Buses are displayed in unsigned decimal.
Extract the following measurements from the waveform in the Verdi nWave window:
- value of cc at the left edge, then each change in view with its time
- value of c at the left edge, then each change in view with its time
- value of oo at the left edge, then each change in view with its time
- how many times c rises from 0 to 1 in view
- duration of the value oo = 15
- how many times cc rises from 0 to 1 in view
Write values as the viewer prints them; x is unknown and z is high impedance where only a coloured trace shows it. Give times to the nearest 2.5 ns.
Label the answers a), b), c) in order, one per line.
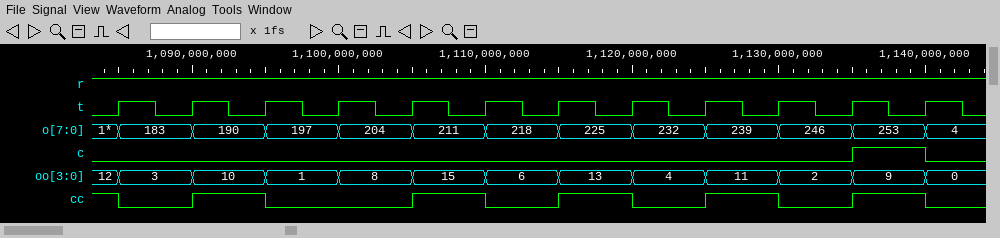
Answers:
a) 1, 0 at 1085 ns, 1 at 1090 ns, 0 at 1095 ns, 1 at 1105 ns, 0 at 1110 ns, 1 at 1115 ns, 0 at 1120 ns, 1 at 1125 ns, 0 at 1130 ns, 1 at 1135 ns, 0 at 1140 ns
b) 0, 1 at 1135 ns, 0 at 1140 ns
c) 12, 3 at 1085 ns, 10 at 1090 ns, 1 at 1095 ns, 8 at 1100 ns, 15 at 1105 ns, 6 at 1110 ns, 13 at 1115 ns, 4 at 1120 ns, 11 at 1125 ns, 2 at 1130 ns, 9 at 1135 ns, 0 at 1140 ns
d) 1
e) 5 ns
f) 5
